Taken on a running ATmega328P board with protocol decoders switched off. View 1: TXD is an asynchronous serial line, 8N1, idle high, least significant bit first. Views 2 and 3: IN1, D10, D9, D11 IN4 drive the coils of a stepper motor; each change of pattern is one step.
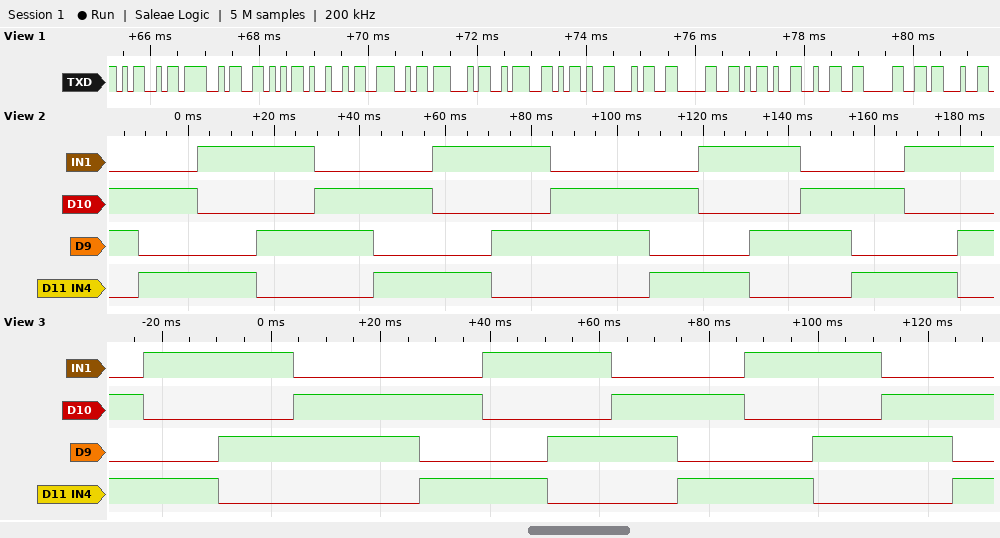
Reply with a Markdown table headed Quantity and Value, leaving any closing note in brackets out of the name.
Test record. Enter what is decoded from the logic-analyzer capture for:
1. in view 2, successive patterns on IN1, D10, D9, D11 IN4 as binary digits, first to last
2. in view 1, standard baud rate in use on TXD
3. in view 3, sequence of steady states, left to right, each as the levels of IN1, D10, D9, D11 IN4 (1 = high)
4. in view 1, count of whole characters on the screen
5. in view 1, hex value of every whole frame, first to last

| Quantity | Value |
|---|---|
| in view 2, successive patterns on IN1, D10, D9, D11 IN4 as binary digits, first to last | 0110 0101 1001 1010 0110 0101 1001 1010 0110 0101 1001 1010 0110 0101 1001 1010 |
| in view 1, standard baud rate in use on TXD | 9600 baud |
| in view 3, sequence of steady states, left to right, each as the levels of IN1, D10, D9, D11 IN4 | 0101 1001 1010 0110 0101 1001 1010 0110 0101 1001 1010 0110 0101 |
| in view 1, count of whole characters on the screen | 14 |
| in view 1, hex value of every whole frame, first to last | 4D 4F 56 49 4E 47 3A 2D 34 30 2D 32 30 23 |
